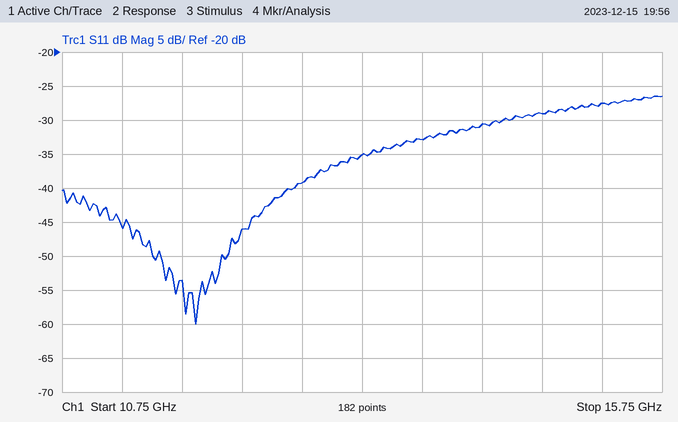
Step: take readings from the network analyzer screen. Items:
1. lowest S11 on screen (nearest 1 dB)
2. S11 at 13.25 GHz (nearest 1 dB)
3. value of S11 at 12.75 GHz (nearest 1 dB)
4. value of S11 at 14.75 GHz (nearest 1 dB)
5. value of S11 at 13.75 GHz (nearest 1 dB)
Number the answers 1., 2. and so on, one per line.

1. -60 dB
2. -35 dB
3. -39 dB
4. -29 dB
5. -33 dB
